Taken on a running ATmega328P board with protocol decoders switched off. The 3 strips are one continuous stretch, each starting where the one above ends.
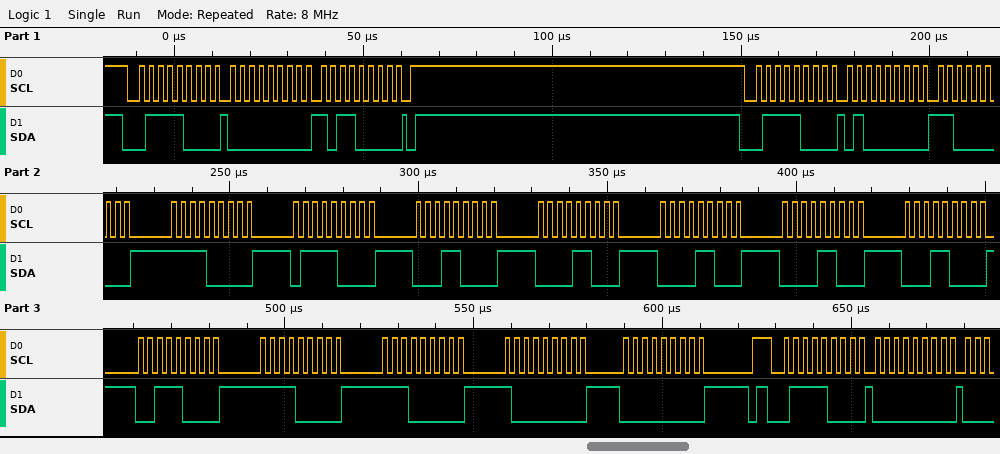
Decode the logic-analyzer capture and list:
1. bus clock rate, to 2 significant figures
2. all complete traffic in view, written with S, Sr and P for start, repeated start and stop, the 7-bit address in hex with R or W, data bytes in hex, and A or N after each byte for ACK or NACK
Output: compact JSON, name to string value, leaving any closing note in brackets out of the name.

{"bus clock rate, to 2 significant figures": "400 kHz", "all complete traffic in view, written with S, Sr and P for start, repeated start and stop, the 7-bit address in hex with R or W, data bytes in hex, and A or N after each byte for ACK or NACK": "S 3CW A 00 A B0 A P S 3CW A 40 A C0 A F0 A 78 A 18 A 0C A 0C A 0C A 18 A 38 A F0 A E0 A 80 A 00 A P S 3CW A 00 A"}
